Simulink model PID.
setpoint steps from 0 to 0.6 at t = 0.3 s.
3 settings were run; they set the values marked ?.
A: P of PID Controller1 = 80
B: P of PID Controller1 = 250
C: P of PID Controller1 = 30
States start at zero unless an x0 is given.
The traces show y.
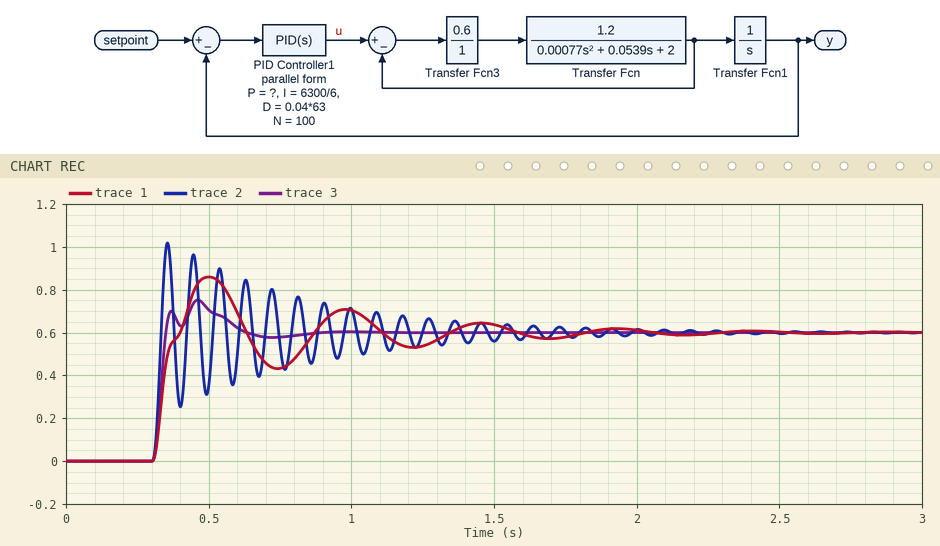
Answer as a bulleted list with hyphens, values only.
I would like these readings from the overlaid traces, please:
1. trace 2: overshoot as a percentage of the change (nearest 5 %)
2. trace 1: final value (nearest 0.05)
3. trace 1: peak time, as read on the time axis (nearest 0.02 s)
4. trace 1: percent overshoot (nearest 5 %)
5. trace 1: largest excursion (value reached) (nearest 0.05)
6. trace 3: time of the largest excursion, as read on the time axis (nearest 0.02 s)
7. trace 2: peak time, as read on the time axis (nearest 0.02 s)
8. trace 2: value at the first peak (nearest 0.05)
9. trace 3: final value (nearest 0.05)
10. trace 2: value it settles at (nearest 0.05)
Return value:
- 70 %
- 0.60
- 0.50 s
- 45 %
- 0.85
- 0.46 s
- 0.36 s
- 1.00
- 0.60
- 0.60
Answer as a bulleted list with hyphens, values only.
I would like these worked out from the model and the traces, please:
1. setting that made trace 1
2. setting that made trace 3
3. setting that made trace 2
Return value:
- C
- A
- B
